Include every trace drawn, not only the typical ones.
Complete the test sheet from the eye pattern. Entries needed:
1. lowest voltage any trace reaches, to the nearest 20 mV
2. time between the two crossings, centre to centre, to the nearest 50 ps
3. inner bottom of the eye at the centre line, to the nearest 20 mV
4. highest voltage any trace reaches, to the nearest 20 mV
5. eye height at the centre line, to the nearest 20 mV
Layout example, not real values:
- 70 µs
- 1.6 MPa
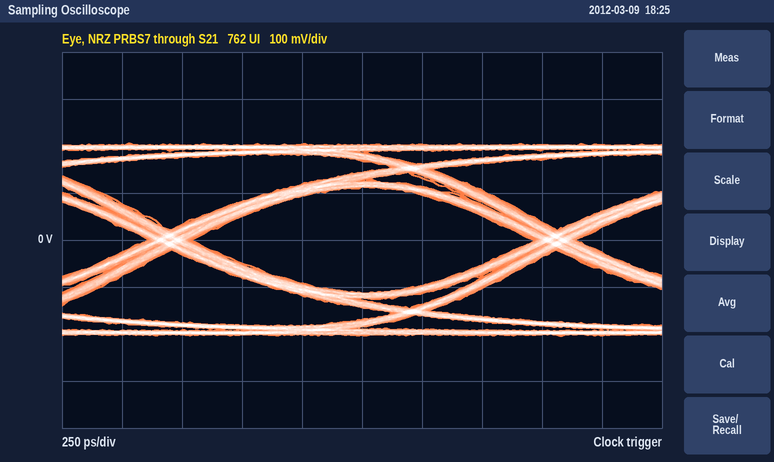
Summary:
- -200 mV
- 1.60 ns
- -120 mV
- 200 mV
- 220 mV
